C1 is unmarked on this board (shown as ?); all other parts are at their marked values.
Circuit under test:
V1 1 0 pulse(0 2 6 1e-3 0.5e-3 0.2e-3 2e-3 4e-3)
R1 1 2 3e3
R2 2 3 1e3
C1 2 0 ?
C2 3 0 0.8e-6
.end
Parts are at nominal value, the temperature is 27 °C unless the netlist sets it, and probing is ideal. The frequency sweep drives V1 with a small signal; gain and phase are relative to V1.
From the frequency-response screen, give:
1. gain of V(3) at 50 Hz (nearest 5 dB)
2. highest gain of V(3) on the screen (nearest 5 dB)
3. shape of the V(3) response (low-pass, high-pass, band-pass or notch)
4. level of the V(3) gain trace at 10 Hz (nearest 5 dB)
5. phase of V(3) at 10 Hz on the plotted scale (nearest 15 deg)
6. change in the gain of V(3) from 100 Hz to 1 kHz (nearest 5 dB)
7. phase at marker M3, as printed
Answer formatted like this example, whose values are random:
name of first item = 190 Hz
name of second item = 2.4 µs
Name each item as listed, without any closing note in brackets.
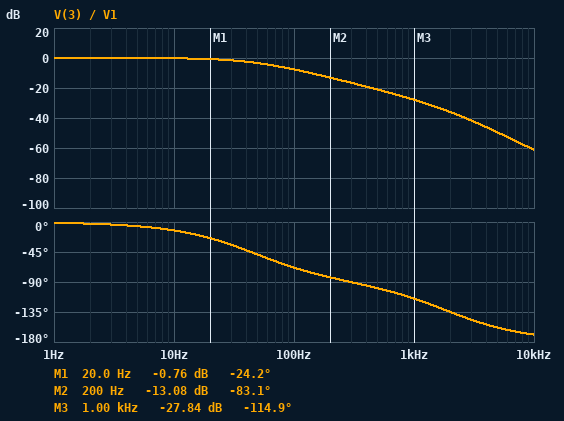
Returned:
gain of V(3) at 50 Hz = -5 dB
highest gain of V(3) on the screen = 0 dB
shape of the V(3) response = low-pass
level of the V(3) gain trace at 10 Hz = 0 dB
phase of V(3) at 10 Hz on the plotted scale = -15 deg
change in the gain of V(3) from 100 Hz to 1 kHz = -20 dB
phase at marker M3, as printed = -114.9 deg
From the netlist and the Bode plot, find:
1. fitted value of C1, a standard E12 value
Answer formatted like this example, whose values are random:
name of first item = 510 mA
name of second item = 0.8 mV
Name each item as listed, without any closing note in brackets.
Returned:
fitted value of C1, a standard E12 value = 120 nF
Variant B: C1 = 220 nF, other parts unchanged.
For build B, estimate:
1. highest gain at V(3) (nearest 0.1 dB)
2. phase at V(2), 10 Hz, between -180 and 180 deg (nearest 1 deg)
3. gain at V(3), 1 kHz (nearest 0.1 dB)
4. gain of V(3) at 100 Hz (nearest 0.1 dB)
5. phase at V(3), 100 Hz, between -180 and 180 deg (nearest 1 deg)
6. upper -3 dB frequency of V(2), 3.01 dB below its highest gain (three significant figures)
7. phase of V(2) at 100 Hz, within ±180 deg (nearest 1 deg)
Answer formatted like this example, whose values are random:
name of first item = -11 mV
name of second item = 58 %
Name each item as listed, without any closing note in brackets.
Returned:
highest gain at V(3) = 0 dB
phase at V(2), 10 Hz, between -180 and 180 deg = -11 deg
gain at V(3), 1 kHz = -29.9 dB
gain of V(3) at 100 Hz = -8.1 dB
phase at V(3), 100 Hz, between -180 and 180 deg = -72 deg
upper -3 dB frequency of V(2), 3.01 dB below its highest gain = 44.9 Hz
phase of V(2) at 100 Hz, within ±180 deg = -45 deg
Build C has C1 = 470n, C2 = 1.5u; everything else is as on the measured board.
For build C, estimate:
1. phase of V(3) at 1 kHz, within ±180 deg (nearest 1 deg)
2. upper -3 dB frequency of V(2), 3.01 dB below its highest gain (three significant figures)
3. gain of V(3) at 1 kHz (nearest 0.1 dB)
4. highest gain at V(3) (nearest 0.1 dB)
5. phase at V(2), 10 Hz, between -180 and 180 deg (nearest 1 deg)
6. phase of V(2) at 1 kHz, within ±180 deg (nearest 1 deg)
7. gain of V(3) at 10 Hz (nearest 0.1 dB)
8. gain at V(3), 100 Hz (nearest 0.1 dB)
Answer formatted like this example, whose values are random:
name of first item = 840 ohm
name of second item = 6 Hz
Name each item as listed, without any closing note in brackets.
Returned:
phase of V(3) at 1 kHz, within ±180 deg = -151 deg
upper -3 dB frequency of V(2), 3.01 dB below its highest gain = 23.4 Hz
gain of V(3) at 1 kHz = -39.5 dB
highest gain at V(3) = 0 dB
phase at V(2), 10 Hz, between -180 and 180 deg = -20 deg
phase of V(2) at 1 kHz, within ±180 deg = -67 deg
gain of V(3) at 10 Hz = -0.8 dB
gain at V(3), 100 Hz = -13.4 dB
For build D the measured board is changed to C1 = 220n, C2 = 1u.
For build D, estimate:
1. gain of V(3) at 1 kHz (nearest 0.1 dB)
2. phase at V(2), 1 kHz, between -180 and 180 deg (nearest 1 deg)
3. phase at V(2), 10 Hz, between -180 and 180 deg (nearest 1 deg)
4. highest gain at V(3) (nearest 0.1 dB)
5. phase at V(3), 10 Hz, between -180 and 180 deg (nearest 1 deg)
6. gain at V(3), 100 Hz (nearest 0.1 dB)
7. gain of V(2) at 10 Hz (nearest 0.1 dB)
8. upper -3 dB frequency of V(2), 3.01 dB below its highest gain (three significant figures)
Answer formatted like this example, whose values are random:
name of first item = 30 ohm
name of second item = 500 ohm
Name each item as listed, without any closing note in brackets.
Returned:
gain of V(3) at 1 kHz = -31.7 dB
phase at V(2), 1 kHz, between -180 and 180 deg = -50 deg
phase at V(2), 10 Hz, between -180 and 180 deg = -13 deg
highest gain at V(3) = 0 dB
phase at V(3), 10 Hz, between -180 and 180 deg = -16 deg
gain at V(3), 100 Hz = -9.6 dB
gain of V(2) at 10 Hz = -0.3 dB
upper -3 dB frequency of V(2), 3.01 dB below its highest gain = 37.1 Hz
